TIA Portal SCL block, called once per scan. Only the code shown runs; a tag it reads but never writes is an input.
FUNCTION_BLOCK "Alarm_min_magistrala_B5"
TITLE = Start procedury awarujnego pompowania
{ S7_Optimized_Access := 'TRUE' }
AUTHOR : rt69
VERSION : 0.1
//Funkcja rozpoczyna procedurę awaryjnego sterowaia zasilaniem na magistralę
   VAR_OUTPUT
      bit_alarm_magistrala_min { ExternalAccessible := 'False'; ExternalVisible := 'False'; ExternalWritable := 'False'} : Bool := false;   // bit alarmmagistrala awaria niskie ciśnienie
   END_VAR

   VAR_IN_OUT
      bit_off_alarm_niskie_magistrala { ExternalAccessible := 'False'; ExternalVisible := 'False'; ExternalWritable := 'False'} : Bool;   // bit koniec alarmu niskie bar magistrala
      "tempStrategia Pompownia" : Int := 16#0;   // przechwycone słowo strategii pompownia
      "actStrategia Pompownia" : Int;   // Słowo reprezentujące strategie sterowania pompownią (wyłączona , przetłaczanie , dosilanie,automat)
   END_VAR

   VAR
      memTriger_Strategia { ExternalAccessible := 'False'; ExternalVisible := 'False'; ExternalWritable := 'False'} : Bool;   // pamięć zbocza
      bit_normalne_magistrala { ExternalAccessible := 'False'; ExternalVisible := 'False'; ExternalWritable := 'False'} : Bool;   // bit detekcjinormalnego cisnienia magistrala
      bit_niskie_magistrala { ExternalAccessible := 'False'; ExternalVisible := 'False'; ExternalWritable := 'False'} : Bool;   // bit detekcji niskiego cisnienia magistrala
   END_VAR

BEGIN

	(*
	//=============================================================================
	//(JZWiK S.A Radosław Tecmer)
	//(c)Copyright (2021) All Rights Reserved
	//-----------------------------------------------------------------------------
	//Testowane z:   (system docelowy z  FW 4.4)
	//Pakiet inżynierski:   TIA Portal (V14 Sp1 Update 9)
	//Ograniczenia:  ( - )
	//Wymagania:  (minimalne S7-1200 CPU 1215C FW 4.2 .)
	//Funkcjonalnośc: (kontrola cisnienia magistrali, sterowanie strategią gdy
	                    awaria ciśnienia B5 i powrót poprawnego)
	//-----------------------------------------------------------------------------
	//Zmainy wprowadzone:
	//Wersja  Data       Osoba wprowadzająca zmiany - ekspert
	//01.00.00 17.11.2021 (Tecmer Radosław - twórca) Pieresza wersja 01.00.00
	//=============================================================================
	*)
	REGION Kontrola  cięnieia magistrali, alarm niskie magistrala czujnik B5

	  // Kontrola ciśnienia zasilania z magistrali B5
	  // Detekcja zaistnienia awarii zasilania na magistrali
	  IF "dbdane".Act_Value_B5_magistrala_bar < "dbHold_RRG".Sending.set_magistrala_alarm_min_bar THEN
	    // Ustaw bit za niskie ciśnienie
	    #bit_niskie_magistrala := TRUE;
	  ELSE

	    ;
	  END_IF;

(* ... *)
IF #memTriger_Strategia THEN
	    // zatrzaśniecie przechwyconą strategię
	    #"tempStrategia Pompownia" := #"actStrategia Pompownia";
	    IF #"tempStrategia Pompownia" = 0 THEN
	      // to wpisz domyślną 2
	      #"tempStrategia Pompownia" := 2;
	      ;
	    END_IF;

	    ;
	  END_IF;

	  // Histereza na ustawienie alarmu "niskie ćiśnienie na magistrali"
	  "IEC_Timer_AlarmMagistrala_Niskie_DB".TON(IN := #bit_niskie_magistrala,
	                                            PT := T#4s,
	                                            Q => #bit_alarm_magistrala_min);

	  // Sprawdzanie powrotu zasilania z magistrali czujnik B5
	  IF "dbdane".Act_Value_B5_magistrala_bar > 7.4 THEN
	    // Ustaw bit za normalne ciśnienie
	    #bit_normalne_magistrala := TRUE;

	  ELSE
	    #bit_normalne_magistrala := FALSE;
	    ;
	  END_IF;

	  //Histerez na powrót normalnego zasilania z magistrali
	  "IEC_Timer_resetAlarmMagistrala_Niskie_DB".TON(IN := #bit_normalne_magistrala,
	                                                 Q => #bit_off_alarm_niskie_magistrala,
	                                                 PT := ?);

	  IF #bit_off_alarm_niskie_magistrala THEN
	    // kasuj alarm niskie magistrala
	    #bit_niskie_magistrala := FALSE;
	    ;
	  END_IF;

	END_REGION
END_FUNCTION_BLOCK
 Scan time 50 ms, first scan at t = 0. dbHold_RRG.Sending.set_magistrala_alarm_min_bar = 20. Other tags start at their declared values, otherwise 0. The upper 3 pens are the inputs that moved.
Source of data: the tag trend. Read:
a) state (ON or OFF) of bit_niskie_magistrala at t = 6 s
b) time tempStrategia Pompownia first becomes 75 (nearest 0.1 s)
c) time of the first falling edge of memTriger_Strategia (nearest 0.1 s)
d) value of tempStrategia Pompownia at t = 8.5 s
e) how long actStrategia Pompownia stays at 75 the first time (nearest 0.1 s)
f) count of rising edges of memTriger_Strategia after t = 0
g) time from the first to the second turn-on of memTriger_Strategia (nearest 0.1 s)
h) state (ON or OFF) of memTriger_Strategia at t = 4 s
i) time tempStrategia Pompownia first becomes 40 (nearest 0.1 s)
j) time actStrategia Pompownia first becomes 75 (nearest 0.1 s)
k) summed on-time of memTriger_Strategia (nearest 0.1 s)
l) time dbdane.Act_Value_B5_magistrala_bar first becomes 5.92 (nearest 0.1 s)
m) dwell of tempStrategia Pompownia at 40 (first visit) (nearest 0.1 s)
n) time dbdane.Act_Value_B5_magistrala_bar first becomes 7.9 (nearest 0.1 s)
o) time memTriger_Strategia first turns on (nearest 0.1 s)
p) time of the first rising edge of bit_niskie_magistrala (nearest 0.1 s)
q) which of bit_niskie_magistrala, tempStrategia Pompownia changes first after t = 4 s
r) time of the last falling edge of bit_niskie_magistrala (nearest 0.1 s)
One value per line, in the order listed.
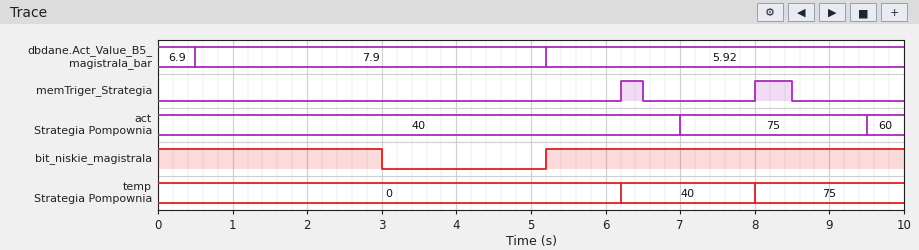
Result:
ON
8.0 s
6.5 s
75
2.5 s
2
1.8 s
OFF
6.2 s
7.0 s
0.8 s
5.2 s
1.8 s
0.5 s
6.2 s
5.2 s
bit_niskie_magistrala
3.0 s
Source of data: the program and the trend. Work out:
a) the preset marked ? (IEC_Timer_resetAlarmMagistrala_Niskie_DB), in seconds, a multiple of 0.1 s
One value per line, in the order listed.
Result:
2.5 s
